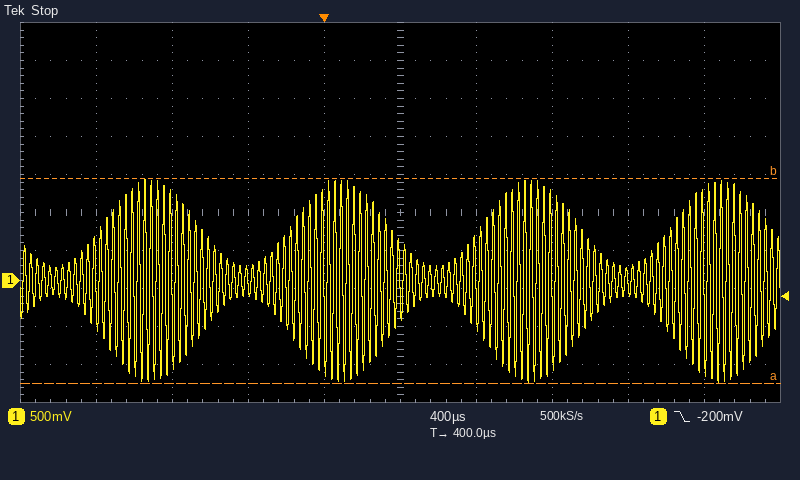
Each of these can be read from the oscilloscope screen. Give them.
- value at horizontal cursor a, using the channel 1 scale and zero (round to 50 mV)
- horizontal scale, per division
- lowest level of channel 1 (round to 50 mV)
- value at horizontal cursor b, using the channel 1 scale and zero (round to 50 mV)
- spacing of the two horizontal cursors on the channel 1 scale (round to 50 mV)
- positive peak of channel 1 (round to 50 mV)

-1.35 V
400 µs
-1.35 V
1.35 V
2.70 V
1.35 V
